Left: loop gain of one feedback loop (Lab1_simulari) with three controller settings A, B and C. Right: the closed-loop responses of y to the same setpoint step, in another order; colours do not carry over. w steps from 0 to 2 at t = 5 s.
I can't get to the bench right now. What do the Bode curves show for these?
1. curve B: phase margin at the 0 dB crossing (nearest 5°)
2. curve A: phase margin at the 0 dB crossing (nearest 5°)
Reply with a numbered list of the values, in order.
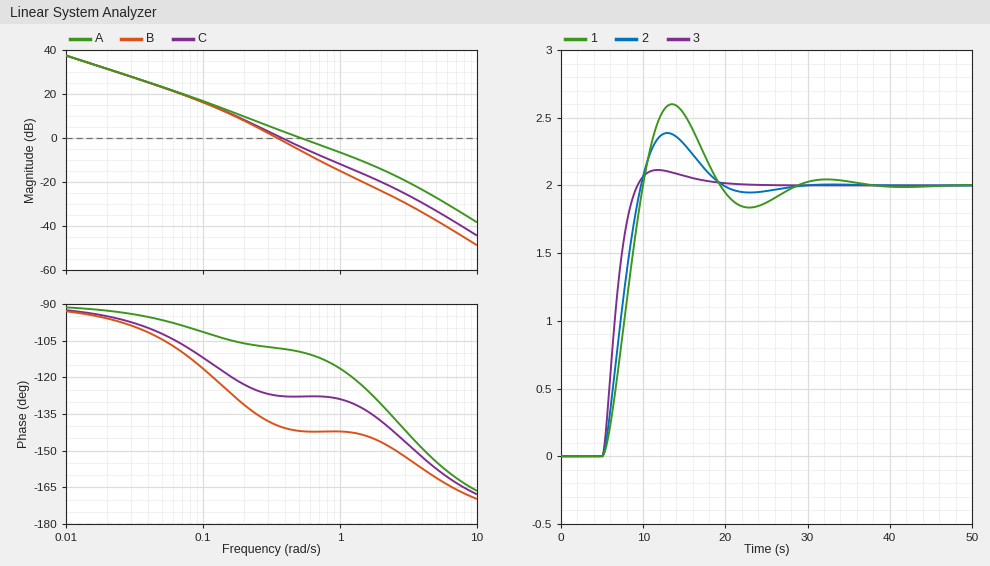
1. 40°
2. 70°
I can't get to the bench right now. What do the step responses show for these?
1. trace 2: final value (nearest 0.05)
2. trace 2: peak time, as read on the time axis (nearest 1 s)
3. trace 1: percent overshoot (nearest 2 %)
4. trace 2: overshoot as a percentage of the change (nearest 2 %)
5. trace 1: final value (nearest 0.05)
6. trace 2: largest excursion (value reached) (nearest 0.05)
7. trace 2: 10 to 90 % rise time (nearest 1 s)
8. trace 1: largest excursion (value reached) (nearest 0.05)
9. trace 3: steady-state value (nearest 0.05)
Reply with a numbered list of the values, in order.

1. 2.00
2. 13 s
3. 30 %
4. 20 %
5. 2.00
6. 2.40
7. 3 s
8. 2.60
9. 2.00
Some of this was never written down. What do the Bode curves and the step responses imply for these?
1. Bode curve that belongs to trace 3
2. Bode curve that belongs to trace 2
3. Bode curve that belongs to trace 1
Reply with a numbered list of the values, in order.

1. A
2. C
3. B
